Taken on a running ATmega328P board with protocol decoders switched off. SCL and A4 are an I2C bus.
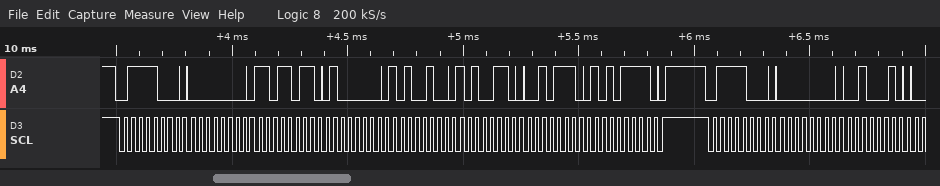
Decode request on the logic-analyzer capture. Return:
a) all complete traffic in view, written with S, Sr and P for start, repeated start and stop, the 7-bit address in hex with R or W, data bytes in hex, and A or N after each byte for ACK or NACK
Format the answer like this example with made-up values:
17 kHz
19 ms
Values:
S 3CW A 00 A DB A 40 A A4 A A6 A 2E A AF A P S 3CW A 00 A 22 A
